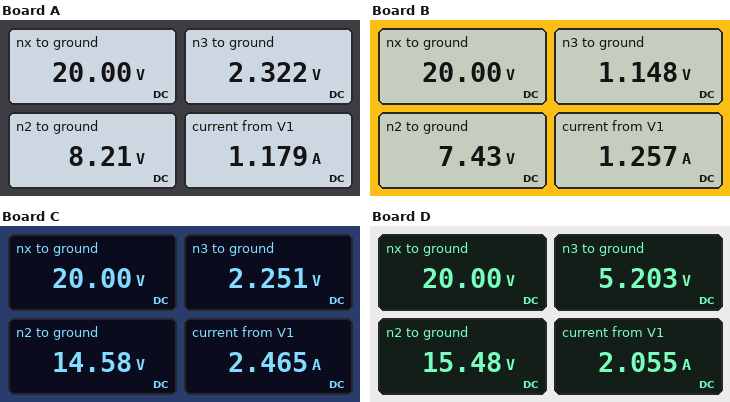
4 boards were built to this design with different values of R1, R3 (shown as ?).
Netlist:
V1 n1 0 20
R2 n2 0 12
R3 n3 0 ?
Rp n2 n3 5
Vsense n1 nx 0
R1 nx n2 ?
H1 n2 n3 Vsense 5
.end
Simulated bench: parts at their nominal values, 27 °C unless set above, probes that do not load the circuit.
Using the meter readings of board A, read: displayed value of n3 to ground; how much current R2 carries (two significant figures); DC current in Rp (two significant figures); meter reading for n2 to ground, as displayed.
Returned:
2.322 V
680 mA
1.2 A
8.21 V
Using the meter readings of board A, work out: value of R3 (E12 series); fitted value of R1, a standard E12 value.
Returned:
4.7 Ω
10 Ω
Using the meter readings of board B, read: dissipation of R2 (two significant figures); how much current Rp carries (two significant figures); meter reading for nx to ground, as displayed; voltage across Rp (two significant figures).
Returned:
4.6 W
1.3 A
20.00 V
6.3 V
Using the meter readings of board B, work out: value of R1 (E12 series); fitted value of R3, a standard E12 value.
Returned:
10 Ω
1.8 Ω
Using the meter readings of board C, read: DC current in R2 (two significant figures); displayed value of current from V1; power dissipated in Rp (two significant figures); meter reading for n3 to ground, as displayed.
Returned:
1.2 A
2.465 A
30 W
2.251 V
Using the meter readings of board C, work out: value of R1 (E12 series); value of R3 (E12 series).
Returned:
2.2 Ω
1.8 Ω
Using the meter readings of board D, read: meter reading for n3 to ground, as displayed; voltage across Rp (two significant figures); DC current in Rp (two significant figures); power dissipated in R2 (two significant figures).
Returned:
5.203 V
10 V
2.1 A
20 W
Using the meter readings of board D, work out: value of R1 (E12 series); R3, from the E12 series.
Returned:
2.2 Ω
6.8 Ω
